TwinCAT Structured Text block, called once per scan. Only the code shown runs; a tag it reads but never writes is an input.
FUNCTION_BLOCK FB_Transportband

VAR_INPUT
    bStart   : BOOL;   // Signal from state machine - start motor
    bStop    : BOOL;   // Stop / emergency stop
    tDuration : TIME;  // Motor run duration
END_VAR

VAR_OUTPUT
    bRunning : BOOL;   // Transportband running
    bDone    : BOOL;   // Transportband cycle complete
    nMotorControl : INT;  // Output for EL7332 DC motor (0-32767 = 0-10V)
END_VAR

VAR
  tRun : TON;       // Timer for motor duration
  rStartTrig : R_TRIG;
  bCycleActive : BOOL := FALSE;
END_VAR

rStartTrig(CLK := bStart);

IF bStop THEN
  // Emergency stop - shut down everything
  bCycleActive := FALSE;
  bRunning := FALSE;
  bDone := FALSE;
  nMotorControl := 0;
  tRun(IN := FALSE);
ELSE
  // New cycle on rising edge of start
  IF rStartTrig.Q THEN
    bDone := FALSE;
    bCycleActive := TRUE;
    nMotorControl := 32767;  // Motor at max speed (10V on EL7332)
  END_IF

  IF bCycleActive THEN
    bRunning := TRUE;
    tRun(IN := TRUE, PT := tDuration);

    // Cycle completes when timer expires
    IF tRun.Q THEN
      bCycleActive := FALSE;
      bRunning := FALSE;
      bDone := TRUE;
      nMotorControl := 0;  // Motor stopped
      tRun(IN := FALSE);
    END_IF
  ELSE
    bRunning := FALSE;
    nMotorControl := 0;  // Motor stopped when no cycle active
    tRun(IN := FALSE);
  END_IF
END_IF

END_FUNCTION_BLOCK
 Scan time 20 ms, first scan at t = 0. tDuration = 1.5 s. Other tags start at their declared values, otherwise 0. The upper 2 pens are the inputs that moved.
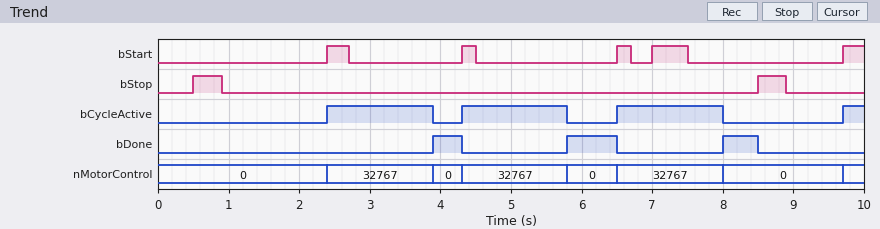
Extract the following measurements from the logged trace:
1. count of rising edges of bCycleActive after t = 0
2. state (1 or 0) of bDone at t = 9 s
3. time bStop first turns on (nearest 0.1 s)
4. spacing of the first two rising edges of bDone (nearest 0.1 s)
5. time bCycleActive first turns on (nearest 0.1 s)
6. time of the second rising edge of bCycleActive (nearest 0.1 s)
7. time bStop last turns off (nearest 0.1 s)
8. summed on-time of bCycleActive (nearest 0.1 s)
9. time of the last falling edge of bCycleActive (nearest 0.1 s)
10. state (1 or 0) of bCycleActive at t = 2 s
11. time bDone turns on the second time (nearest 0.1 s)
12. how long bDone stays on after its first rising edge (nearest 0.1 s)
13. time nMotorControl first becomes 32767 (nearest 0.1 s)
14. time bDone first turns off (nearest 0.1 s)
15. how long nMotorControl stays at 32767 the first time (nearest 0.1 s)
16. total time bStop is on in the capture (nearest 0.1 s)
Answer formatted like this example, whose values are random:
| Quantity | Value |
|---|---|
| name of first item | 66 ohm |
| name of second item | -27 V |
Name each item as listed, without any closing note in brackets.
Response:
| Quantity | Value |
|---|---|
| count of rising edges of bCycleActive after t = 0 | 4 |
| state (1 or 0) of bDone at t = 9 s | 0 |
| time bStop first turns on | 0.5 s |
| spacing of the first two rising edges of bDone | 1.9 s |
| time bCycleActive first turns on | 2.4 s |
| time of the second rising edge of bCycleActive | 4.3 s |
| time bStop last turns off | 8.9 s |
| summed on-time of bCycleActive | 4.8 s |
| time of the last falling edge of bCycleActive | 8.0 s |
| state (1 or 0) of bCycleActive at t = 2 s | 0 |
| time bDone turns on the second time | 5.8 s |
| how long bDone stays on after its first rising edge | 0.4 s |
| time nMotorControl first becomes 32767 | 2.4 s |
| time bDone first turns off | 4.3 s |
| how long nMotorControl stays at 32767 the first time | 1.5 s |
| total time bStop is on in the capture | 0.8 s |
